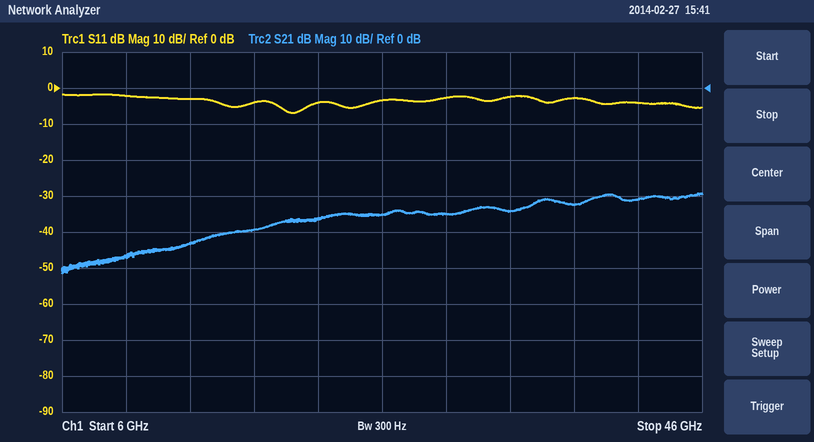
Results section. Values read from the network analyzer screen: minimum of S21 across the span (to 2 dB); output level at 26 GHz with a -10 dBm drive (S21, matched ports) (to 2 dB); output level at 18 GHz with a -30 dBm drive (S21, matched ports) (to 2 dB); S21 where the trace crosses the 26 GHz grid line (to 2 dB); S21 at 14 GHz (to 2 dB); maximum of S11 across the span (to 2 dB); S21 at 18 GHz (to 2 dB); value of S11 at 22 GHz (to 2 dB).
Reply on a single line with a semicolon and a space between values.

-52 dB; -46 dBm; -70 dBm; -36 dB; -44 dB; -2 dB; -40 dB; -4 dB
